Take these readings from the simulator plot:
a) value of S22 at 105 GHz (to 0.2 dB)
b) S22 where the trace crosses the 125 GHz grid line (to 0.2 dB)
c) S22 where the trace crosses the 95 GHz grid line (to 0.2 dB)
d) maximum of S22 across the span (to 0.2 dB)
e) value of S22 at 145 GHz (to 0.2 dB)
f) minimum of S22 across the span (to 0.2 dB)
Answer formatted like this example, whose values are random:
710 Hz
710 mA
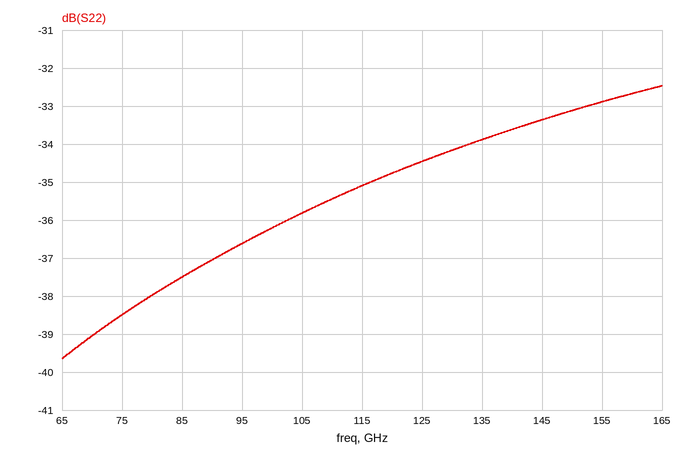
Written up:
-35.8 dB
-34.4 dB
-36.6 dB
-32.4 dB
-33.4 dB
-39.6 dB
